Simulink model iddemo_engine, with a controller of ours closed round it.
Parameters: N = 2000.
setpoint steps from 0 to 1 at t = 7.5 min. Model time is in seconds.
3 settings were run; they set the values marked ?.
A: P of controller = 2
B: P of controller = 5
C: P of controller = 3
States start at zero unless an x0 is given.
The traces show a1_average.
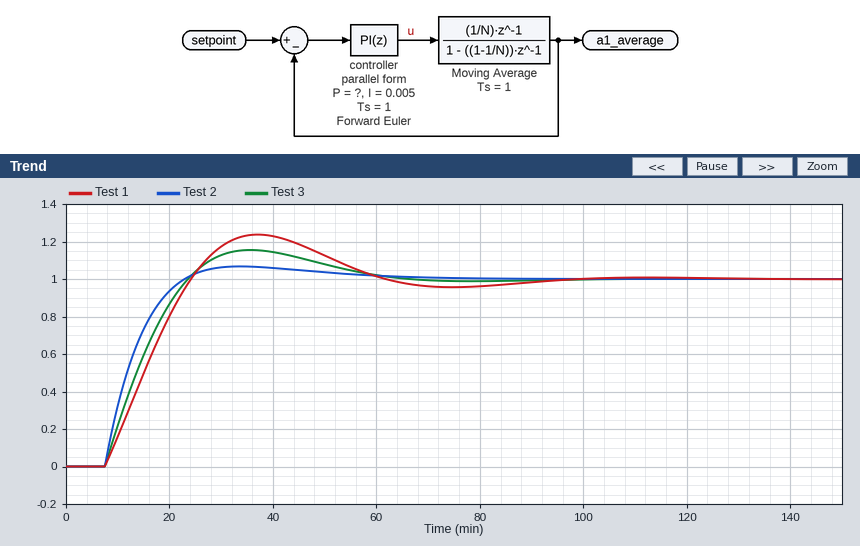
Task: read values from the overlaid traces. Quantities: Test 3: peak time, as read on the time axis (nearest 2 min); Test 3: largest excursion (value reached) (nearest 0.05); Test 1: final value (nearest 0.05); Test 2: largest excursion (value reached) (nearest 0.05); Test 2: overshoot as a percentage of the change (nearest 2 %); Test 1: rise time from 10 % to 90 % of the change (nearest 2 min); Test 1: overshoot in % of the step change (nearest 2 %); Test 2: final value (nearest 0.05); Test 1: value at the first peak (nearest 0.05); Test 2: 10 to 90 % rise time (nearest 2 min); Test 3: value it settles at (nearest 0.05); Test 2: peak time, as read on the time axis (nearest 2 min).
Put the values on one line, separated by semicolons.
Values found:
36 min; 1.15; 1.00; 1.05; 6 %; 12 min; 24 %; 1.00; 1.25; 10 min; 1.00; 34 min
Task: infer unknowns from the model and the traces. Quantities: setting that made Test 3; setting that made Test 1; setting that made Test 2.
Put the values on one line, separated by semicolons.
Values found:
C; A; B
